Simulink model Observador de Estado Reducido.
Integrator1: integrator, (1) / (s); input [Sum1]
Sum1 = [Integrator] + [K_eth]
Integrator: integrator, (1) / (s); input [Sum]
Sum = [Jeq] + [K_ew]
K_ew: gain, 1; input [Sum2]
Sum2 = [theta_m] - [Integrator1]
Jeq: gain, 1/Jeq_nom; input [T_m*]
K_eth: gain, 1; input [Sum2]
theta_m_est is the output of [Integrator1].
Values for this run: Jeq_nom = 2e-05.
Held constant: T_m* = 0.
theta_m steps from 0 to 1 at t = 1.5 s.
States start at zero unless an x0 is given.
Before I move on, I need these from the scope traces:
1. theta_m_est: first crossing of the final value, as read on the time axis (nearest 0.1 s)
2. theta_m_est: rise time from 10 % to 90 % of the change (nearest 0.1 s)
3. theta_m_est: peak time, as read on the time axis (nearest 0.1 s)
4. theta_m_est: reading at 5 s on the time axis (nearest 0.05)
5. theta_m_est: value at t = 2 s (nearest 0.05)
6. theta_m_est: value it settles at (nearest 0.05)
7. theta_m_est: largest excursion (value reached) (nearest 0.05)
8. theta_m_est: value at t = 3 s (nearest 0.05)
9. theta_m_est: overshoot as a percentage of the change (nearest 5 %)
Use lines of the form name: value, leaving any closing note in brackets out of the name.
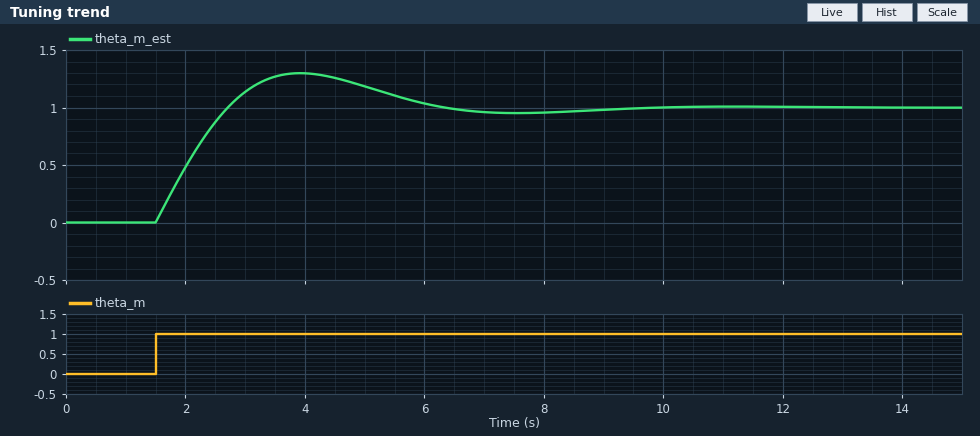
theta_m_est: first crossing of the final value, as read on the time axis: 2.7 s
theta_m_est: rise time from 10 % to 90 % of the change: 0.9 s
theta_m_est: peak time, as read on the time axis: 3.9 s
theta_m_est: reading at 5 s on the time axis: 1.20
theta_m_est: value at t = 2 s: 0.50
theta_m_est: value it settles at: 1.00
theta_m_est: largest excursion (value reached): 1.30
theta_m_est: value at t = 3 s: 1.15
theta_m_est: overshoot as a percentage of the change: 30 %
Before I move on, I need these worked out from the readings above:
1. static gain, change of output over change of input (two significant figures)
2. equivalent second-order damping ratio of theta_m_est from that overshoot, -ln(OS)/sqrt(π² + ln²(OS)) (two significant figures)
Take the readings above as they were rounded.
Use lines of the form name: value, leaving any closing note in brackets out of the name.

static gain, change of output over change of input: 1.0
equivalent second-order damping ratio of theta_m_est from that overshoot, -ln(OS)/sqrt(π² + ln²(OS)): 0.36
